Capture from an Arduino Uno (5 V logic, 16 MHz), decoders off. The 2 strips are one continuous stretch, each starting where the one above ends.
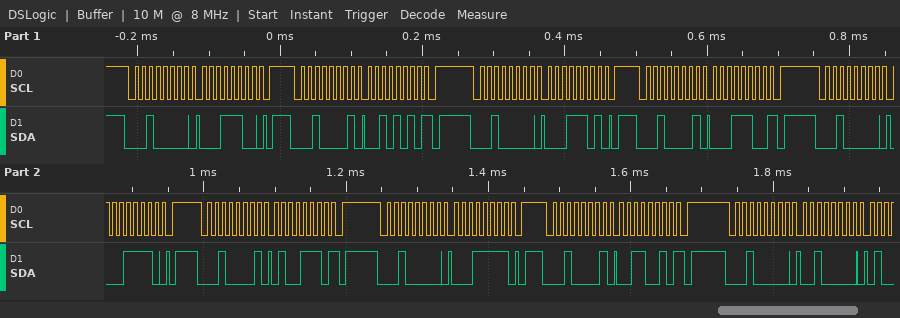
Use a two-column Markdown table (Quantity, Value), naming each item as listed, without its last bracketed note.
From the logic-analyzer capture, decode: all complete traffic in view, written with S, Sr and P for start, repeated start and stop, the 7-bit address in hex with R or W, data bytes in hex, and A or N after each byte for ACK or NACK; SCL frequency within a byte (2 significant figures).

| Quantity | Value |
|---|---|
| all complete traffic in view, written with S, Sr and P for start, repeated start and stop, the 7-bit address in hex with R or W, data bytes in hex, and A or N after each byte for ACK or NACK | S 10W A 1C A P S 10R A 2A N P S 10W A 1D A P S 10R A 1C N P S 10W A 1E A P S 10R A 4E N P S 10W A 1F A P S 10R A 32 N P S 10W A 20 A |
| SCL frequency within a byte | 100 kHz |
